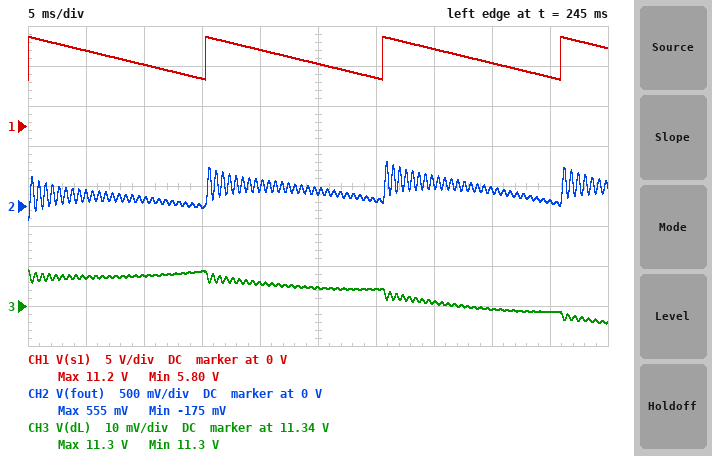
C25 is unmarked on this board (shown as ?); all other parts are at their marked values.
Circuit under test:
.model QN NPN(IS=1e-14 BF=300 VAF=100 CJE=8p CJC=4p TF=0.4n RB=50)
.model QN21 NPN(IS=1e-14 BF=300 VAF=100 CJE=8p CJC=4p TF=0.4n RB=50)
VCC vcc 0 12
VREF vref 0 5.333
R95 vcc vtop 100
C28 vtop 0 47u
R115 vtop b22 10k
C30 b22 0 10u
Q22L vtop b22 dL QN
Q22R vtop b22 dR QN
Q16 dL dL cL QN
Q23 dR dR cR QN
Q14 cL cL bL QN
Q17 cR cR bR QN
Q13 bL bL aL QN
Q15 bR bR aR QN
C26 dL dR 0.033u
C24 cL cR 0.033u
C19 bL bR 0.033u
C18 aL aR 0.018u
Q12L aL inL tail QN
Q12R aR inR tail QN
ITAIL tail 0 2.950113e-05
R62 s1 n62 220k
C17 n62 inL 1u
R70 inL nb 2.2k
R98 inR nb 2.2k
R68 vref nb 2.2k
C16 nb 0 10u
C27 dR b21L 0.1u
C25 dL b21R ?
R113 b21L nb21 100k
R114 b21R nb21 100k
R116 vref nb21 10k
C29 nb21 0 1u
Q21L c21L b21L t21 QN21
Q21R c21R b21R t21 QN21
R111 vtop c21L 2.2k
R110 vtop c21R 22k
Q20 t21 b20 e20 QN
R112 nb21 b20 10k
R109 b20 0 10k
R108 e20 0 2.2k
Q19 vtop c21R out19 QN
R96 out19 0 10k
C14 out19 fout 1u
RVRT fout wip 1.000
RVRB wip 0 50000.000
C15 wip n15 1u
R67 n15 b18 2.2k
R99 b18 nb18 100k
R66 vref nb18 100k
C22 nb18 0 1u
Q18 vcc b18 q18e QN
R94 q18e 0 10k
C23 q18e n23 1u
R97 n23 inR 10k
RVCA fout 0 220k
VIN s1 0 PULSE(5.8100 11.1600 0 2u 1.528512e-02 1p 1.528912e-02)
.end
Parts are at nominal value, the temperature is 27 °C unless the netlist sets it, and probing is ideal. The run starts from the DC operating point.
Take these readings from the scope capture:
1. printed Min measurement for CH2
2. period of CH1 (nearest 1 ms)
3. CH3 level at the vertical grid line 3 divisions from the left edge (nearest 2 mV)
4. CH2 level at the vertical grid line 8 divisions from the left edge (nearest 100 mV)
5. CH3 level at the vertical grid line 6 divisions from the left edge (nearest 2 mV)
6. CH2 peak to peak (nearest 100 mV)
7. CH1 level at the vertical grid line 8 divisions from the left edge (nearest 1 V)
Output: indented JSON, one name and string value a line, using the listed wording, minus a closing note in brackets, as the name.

{
  "printed Min measurement for CH2": "-175 mV",
  "period of CH1": "15 ms",
  "CH3 level at the vertical grid line 3 divisions from the left edge": "11.348 V",
  "CH2 level at the vertical grid line 8 divisions from the left edge": "200 mV",
  "CH3 level at the vertical grid line 6 divisions from the left edge": "11.344 V",
  "CH2 peak to peak": "700 mV",
  "CH1 level at the vertical grid line 8 divisions from the left edge": "8 V"
}
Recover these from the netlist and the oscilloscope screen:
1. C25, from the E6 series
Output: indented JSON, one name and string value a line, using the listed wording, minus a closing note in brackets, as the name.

{
  "C25, from the E6 series": "220 nF"
}
